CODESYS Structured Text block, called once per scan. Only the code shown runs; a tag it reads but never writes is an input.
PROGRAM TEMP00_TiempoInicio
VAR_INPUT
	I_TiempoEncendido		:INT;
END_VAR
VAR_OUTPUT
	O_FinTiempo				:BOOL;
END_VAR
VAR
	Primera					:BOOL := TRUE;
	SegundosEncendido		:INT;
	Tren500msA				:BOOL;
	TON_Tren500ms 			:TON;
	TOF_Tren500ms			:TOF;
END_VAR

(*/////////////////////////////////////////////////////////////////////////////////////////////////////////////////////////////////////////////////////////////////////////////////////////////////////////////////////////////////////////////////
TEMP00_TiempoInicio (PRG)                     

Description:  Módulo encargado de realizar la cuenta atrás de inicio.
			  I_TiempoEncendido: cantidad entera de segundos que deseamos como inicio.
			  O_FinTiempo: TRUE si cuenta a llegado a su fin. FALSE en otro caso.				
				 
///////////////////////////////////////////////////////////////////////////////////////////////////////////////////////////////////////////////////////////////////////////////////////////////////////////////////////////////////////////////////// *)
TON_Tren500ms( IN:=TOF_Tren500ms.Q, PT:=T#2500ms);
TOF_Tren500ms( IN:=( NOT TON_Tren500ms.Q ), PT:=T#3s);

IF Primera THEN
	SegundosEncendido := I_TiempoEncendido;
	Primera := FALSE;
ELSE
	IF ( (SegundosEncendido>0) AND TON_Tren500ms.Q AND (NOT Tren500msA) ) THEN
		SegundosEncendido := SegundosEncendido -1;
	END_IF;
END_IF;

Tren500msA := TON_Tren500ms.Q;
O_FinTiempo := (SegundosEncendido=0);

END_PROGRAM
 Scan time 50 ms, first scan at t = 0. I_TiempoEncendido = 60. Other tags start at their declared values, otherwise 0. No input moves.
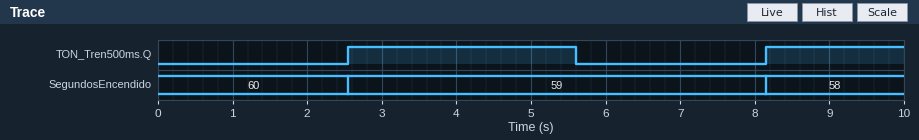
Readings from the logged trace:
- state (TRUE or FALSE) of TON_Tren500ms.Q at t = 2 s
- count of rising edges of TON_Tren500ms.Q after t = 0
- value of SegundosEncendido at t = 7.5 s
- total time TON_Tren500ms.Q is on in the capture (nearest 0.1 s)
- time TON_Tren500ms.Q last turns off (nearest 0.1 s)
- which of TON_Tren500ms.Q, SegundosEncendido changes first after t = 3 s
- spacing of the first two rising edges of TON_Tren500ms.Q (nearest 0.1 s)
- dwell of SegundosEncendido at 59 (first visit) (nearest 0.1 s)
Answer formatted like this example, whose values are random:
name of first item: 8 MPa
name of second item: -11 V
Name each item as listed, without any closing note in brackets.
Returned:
state (TRUE or FALSE) of TON_Tren500ms.Q at t = 2 s: FALSE
count of rising edges of TON_Tren500ms.Q after t = 0: 2
value of SegundosEncendido at t = 7.5 s: 59
total time TON_Tren500ms.Q is on in the capture: 4.9 s
time TON_Tren500ms.Q last turns off: 5.6 s
which of TON_Tren500ms.Q, SegundosEncendido changes first after t = 3 s: TON_Tren500ms.Q
spacing of the first two rising edges of TON_Tren500ms.Q: 5.6 s
dwell of SegundosEncendido at 59 (first visit): 5.6 s
